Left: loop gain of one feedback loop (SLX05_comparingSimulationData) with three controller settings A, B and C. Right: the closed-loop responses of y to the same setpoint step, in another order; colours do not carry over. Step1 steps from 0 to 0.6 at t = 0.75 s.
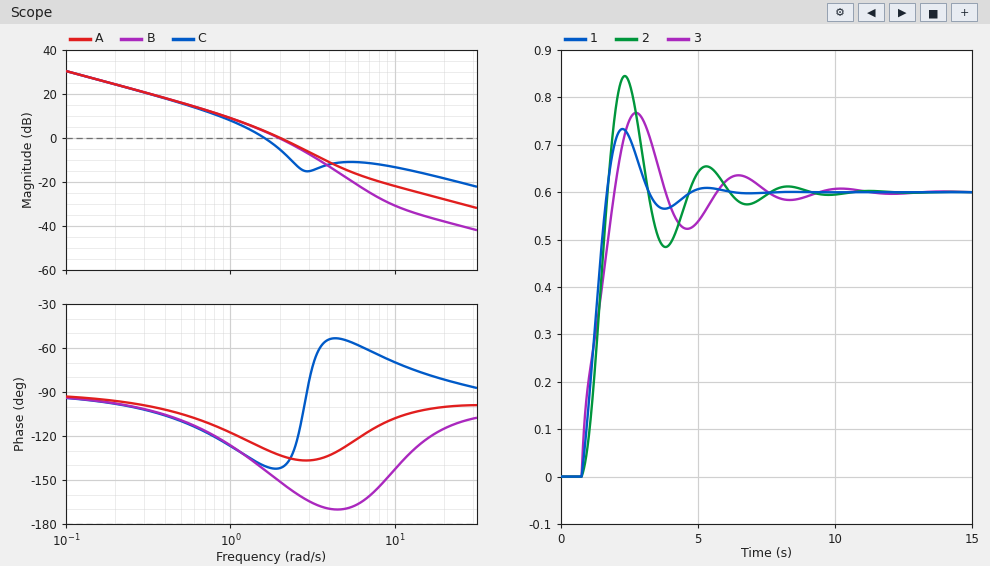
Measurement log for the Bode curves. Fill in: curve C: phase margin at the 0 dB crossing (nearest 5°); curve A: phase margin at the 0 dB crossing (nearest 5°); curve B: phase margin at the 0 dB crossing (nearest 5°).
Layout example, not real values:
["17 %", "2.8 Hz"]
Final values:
["40°", "45°", "30°"]
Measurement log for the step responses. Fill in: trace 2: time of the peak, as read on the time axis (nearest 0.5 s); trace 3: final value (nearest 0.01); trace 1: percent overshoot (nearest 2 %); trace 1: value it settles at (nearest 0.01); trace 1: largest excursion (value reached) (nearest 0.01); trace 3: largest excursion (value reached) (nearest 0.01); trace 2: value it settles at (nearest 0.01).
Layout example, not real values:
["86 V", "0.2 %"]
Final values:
["2.5 s", "0.60", "22 %", "0.60", "0.73", "0.77", "0.60"]
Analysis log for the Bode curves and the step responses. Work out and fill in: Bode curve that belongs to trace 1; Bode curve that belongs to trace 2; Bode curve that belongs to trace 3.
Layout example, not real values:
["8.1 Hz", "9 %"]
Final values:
["A", "B", "C"]
